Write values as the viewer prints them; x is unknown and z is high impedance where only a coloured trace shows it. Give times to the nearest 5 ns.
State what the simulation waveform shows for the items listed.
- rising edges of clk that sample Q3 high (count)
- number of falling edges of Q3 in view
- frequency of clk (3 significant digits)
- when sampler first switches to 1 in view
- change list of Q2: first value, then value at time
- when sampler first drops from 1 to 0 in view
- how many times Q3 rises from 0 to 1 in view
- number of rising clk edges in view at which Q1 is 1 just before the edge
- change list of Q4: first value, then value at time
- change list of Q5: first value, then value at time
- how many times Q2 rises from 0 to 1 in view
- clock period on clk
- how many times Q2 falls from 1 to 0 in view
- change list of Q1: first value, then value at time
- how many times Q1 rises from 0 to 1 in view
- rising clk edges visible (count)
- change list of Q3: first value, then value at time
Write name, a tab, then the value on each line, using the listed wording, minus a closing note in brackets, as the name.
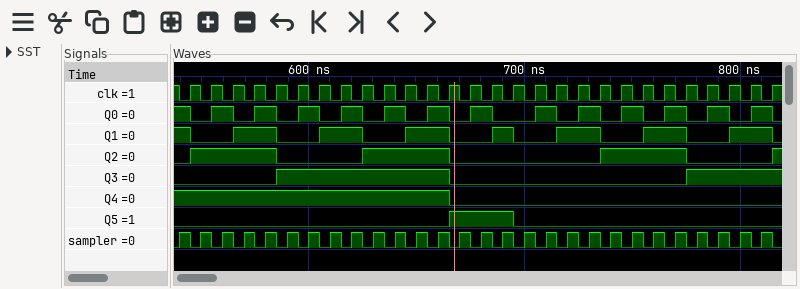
rising edges of clk that sample Q3 high	12
number of falling edges of Q3 in view	1
frequency of clk	100 MHz
when sampler first switches to 1 in view	540 ns
change list of Q2: first value, then value at time	0, 1 at 545 ns, 0 at 585 ns, 1 at 625 ns, 0 at 665 ns, 1 at 735 ns, 0 at 775 ns, 1 at 815 ns
when sampler first drops from 1 to 0 in view	545 ns
how many times Q3 rises from 0 to 1 in view	2
number of rising clk edges in view at which Q1 is 1 just before the edge	14
change list of Q4: first value, then value at time	1, 0 at 665 ns
change list of Q5: first value, then value at time	0, 1 at 665 ns, 0 at 695 ns
how many times Q2 rises from 0 to 1 in view	4
clock period on clk	10 ns
how many times Q2 falls from 1 to 0 in view	3
change list of Q1: first value, then value at time	1, 0 at 545 ns, 1 at 565 ns, 0 at 585 ns, 1 at 605 ns, 0 at 625 ns, 1 at 645 ns, 0 at 665 ns, 1 at 685 ns, 0 at 695 ns, 1 at 715 ns, 0 at 735 ns, 1 at 755 ns, 0 at 775 ns, 1 at 795 ns, 0 at 815 ns
how many times Q1 rises from 0 to 1 in view	7
rising clk edges visible	28
change list of Q3: first value, then value at time	0, 1 at 585 ns, 0 at 665 ns, 1 at 775 ns
